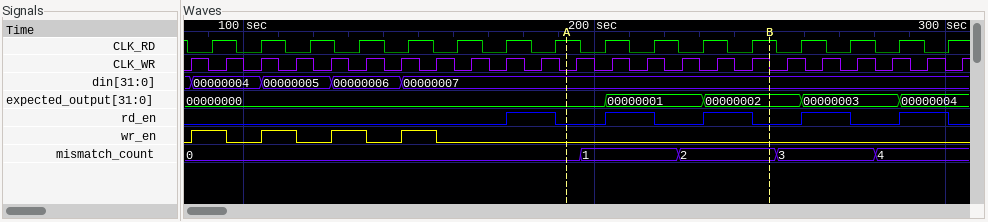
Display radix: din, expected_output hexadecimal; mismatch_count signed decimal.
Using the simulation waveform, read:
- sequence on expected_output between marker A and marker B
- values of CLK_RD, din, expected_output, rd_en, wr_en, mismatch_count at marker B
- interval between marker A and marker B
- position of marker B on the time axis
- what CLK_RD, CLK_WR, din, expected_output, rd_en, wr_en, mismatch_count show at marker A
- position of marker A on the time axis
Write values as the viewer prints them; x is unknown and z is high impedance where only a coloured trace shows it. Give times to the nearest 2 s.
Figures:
00000000, 00000001, 00000002
CLK_RD=1, din=00000007, expected_output=00000002, rd_en=0, wr_en=0, mismatch_count=2
58 s
250 s
CLK_RD=1, CLK_WR=0, din=00000007, expected_output=00000000, rd_en=0, wr_en=0, mismatch_count=0
192 s
